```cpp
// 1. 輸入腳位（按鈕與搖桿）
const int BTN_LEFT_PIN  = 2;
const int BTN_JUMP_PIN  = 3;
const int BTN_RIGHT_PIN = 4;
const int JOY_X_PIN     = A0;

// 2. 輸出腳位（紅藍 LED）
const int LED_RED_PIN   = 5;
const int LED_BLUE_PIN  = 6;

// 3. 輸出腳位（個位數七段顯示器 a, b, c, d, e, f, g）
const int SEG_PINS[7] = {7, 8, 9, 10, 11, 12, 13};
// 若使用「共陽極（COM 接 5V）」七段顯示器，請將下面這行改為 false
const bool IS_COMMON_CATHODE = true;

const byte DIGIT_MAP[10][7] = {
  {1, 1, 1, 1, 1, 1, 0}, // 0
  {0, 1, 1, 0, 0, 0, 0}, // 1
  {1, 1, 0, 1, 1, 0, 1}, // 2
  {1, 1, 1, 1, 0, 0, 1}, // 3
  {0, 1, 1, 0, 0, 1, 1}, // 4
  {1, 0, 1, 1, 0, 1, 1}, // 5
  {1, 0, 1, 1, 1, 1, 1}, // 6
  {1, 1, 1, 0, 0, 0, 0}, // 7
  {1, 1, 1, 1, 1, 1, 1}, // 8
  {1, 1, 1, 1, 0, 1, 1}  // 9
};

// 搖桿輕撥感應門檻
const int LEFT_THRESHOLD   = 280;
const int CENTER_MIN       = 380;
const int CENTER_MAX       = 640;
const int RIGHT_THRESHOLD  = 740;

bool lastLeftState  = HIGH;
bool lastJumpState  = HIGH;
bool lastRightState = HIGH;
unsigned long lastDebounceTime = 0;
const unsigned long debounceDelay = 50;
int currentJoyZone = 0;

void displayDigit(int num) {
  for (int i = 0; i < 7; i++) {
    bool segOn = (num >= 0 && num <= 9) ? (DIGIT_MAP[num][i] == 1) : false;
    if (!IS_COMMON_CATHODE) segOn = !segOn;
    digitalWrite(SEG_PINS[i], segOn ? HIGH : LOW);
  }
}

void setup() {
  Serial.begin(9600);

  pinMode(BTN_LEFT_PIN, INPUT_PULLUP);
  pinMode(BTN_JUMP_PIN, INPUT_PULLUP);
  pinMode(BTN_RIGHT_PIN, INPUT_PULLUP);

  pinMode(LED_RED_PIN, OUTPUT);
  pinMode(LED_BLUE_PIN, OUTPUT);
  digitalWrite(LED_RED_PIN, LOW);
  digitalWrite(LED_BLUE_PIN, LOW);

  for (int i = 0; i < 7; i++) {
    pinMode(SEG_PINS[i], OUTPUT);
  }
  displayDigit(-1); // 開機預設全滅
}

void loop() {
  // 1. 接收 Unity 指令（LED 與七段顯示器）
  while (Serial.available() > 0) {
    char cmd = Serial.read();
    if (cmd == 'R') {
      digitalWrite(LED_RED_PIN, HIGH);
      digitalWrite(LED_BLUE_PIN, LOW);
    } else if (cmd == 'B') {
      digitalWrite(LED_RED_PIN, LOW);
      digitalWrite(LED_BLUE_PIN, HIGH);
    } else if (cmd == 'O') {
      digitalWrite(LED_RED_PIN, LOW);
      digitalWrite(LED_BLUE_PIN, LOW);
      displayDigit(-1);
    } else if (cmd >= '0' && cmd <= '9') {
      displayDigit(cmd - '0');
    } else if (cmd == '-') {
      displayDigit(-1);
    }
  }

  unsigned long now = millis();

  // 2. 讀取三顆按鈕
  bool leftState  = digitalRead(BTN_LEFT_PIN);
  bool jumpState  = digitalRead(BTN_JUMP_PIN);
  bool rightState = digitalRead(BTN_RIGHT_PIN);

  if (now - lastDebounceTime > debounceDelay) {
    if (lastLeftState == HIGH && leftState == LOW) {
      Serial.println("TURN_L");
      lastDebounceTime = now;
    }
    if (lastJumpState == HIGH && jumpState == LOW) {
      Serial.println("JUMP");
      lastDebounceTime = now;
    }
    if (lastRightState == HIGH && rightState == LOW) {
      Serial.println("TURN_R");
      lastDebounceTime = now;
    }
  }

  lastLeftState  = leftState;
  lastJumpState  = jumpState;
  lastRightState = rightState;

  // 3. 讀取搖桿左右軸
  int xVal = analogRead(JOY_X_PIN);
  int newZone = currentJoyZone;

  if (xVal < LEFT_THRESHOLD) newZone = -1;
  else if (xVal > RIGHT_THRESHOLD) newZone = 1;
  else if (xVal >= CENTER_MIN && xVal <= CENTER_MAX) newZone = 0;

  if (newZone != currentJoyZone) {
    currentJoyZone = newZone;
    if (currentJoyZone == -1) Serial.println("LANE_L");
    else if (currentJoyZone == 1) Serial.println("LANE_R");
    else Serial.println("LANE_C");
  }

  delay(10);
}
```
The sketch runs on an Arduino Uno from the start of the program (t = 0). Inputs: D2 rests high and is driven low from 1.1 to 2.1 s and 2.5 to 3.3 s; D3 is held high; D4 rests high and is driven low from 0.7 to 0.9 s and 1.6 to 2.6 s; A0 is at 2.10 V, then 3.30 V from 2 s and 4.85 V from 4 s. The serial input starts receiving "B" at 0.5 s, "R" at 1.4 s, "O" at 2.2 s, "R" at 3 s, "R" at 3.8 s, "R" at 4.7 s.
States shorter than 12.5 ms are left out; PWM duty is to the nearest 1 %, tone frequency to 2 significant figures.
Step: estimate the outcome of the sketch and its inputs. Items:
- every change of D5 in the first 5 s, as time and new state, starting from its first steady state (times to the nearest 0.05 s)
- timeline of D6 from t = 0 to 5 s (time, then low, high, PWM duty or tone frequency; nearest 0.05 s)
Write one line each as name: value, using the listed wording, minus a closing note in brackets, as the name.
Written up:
every change of D5 in the first 5 s, as time and new state, starting from its first steady state: 0 s low; 1.4 s high; 2.2 s low; 3 s high
timeline of D6 from t = 0 to 5 s: 0 s low; 0.5 s high; 1.4 s low
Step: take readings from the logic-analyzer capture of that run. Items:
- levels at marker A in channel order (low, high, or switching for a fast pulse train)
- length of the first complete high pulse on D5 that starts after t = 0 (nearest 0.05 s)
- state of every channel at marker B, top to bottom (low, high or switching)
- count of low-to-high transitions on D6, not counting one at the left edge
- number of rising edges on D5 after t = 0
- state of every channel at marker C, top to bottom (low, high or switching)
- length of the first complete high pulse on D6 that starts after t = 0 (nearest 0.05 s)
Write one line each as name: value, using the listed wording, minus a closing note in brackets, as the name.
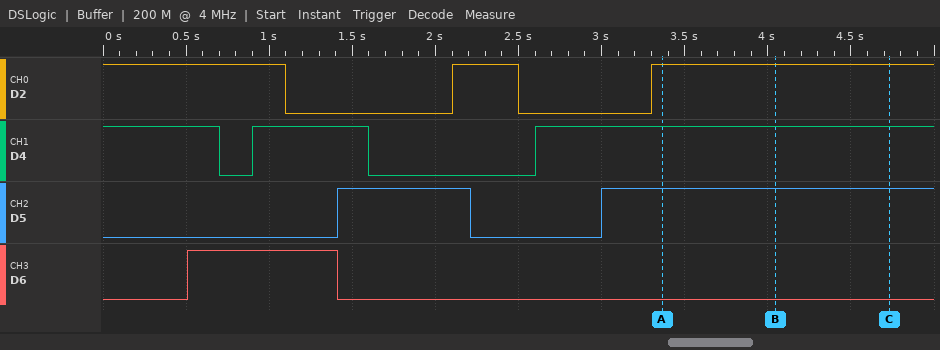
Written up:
levels at marker A in channel order: D2 high, D4 high, D5 high, D6 low
length of the first complete high pulse on D5 that starts after t = 0: 0.80 s
state of every channel at marker B, top to bottom: D2 high, D4 high, D5 high, D6 low
count of low-to-high transitions on D6, not counting one at the left edge: 1
number of rising edges on D5 after t = 0: 2
state of every channel at marker C, top to bottom: D2 high, D4 high, D5 high, D6 low
length of the first complete high pulse on D6 that starts after t = 0: 0.90 s
